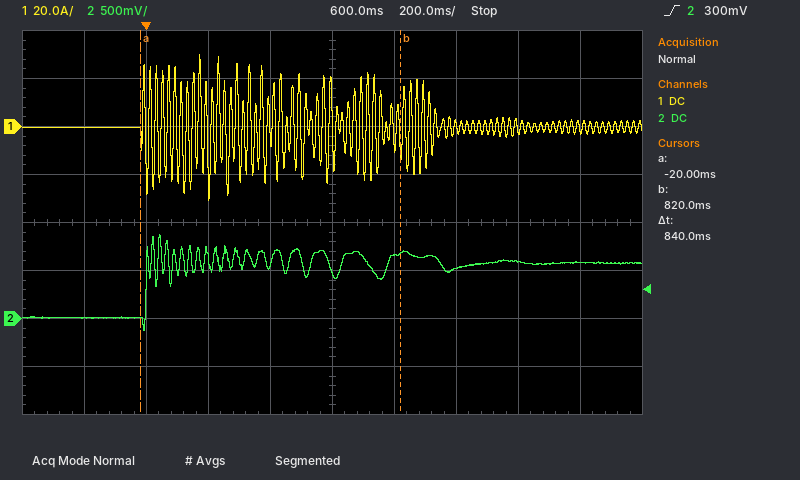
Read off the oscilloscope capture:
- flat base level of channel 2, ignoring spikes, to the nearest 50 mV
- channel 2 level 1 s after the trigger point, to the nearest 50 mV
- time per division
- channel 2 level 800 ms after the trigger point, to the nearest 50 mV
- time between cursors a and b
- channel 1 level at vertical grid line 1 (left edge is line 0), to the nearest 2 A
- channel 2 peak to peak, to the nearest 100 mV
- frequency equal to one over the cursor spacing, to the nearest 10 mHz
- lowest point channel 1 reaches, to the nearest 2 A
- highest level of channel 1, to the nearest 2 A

0 mV
500 mV
200 ms
650 mV
840 ms
0 A
1.00 V
1.19 Hz
-30 A
30 A
